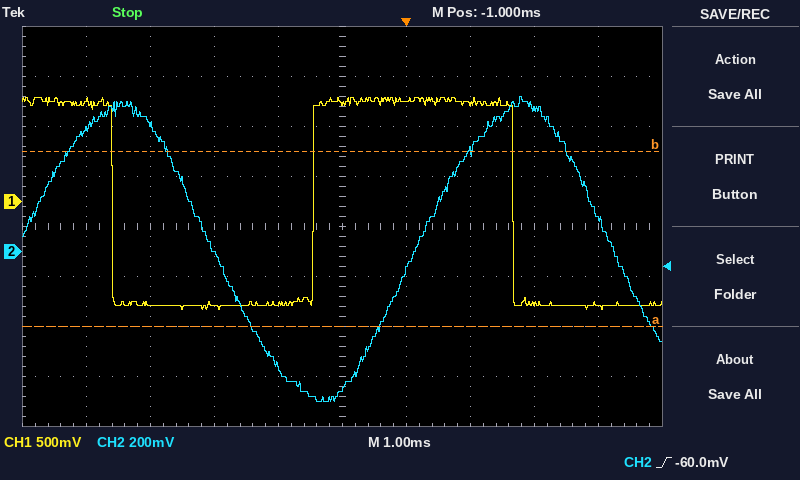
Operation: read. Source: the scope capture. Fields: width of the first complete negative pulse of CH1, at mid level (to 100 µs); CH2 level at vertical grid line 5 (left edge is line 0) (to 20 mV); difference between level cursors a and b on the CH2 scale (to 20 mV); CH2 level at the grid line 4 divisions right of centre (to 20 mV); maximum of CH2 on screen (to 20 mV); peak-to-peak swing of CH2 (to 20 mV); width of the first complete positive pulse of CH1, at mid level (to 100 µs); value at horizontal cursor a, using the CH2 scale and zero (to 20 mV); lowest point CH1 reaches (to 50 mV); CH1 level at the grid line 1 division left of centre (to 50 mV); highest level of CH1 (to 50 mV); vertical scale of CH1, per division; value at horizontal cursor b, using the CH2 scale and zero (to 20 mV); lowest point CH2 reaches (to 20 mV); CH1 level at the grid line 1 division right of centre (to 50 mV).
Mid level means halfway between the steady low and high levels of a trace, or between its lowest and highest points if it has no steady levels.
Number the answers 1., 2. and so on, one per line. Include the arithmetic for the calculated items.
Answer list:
1. 3.1 ms
2. -540 mV
3. 700 mV
4. 140 mV
5. 620 mV
6. 620 mV − (-600 mV) = 1.22 V
7. 3.1 ms
8. -300 mV
9. -1.10 V
10. -1.00 V
11. 1.05 V
12. 500 mV
13. 400 mV
14. -600 mV
15. 1.00 V
